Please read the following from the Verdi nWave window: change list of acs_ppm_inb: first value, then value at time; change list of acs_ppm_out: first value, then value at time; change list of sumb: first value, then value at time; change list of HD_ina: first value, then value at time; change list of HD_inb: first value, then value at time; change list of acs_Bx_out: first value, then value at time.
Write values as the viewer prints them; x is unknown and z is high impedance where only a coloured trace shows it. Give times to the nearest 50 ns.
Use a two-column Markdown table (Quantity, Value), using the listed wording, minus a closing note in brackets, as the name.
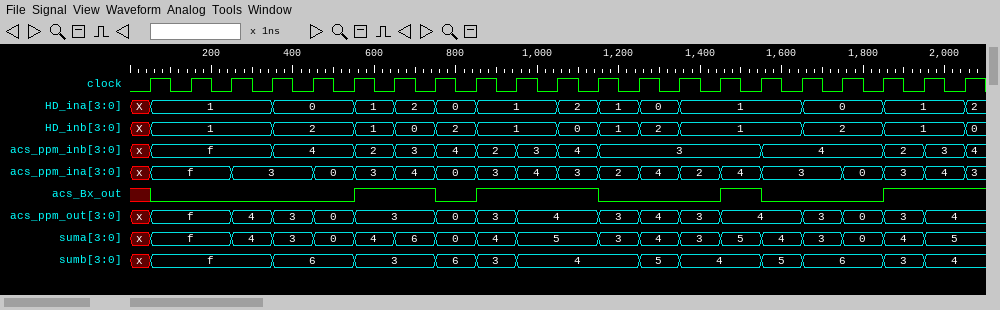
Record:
| Quantity | Value |
|---|---|
| change list of acs_ppm_inb: first value, then value at time | x, f at 50 ns, 4 at 350 ns, 2 at 550 ns, 3 at 650 ns, 4 at 750 ns, 2 at 850 ns, 3 at 950 ns, 4 at 1050 ns, 3 at 1150 ns, 4 at 1550 ns, 2 at 1850 ns, 3 at 1950 ns, 4 at 2050 ns |
| change list of acs_ppm_out: first value, then value at time | x, f at 50 ns, 4 at 250 ns, 3 at 350 ns, 0 at 450 ns, 3 at 550 ns, 0 at 750 ns, 3 at 850 ns, 4 at 950 ns, 3 at 1150 ns, 4 at 1250 ns, 3 at 1350 ns, 4 at 1450 ns, 3 at 1650 ns, 0 at 1750 ns, 3 at 1850 ns, 4 at 1950 ns |
| change list of sumb: first value, then value at time | x, f at 50 ns, 6 at 350 ns, 3 at 550 ns, 6 at 750 ns, 3 at 850 ns, 4 at 950 ns, 5 at 1250 ns, 4 at 1350 ns, 5 at 1550 ns, 6 at 1650 ns, 3 at 1850 ns, 4 at 1950 ns |
| change list of HD_ina: first value, then value at time | X, 1 at 50 ns, 0 at 350 ns, 1 at 550 ns, 2 at 650 ns, 0 at 750 ns, 1 at 850 ns, 2 at 1050 ns, 1 at 1150 ns, 0 at 1250 ns, 1 at 1350 ns, 0 at 1650 ns, 1 at 1850 ns, 2 at 2050 ns |
| change list of HD_inb: first value, then value at time | X, 1 at 50 ns, 2 at 350 ns, 1 at 550 ns, 0 at 650 ns, 2 at 750 ns, 1 at 850 ns, 0 at 1050 ns, 1 at 1150 ns, 2 at 1250 ns, 1 at 1350 ns, 2 at 1650 ns, 1 at 1850 ns, 0 at 2050 ns |
| change list of acs_Bx_out: first value, then value at time | x, 0 at 50 ns, 1 at 550 ns, 0 at 750 ns, 1 at 850 ns, 0 at 1150 ns, 1 at 1450 ns, 0 at 1550 ns, 1 at 1850 ns |
